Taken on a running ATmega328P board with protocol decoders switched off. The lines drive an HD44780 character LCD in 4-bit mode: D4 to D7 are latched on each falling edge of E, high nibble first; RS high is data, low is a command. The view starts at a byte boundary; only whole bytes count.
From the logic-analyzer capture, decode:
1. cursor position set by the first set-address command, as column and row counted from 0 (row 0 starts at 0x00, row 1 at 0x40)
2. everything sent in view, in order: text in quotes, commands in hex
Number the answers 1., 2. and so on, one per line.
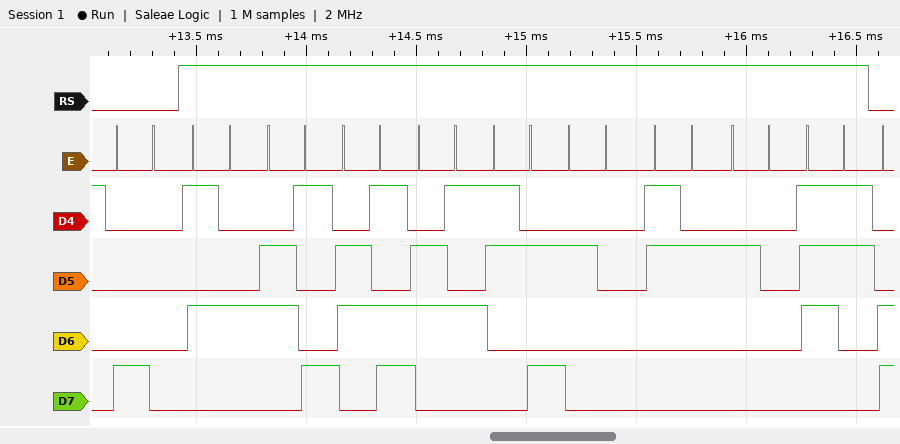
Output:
1. column 0, row 0
2. 0x80 "Time: 2 s"
